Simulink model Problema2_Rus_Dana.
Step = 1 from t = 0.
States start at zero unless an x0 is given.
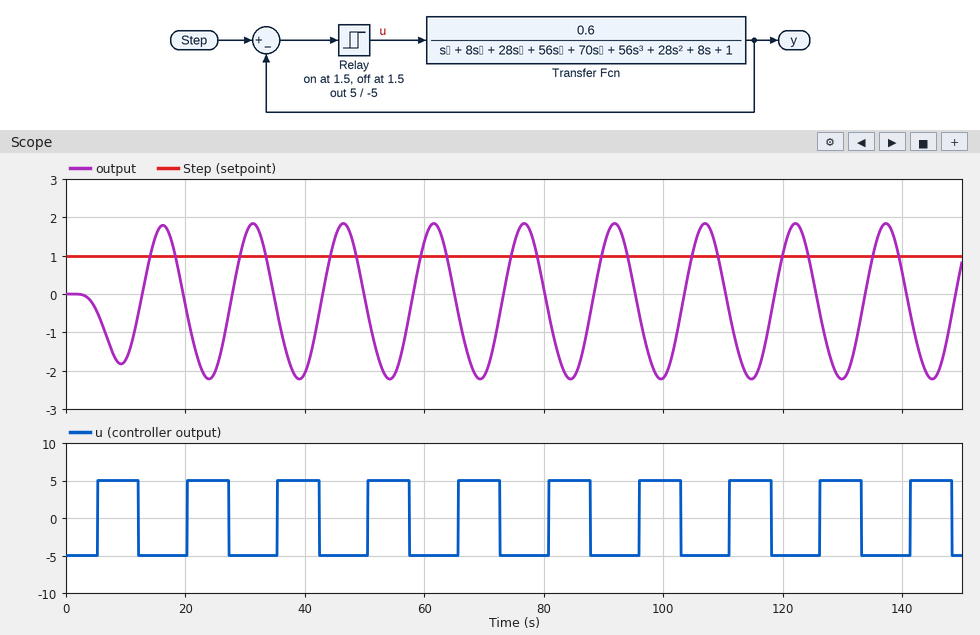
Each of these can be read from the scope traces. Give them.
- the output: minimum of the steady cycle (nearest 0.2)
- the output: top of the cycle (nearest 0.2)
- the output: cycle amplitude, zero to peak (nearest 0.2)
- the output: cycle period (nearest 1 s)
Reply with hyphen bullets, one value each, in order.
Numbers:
- -2.2
- 1.8
- 2.0
- 15 s
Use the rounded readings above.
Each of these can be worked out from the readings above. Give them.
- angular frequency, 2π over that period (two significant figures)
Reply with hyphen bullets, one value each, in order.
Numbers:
- 0.42 rad/s
